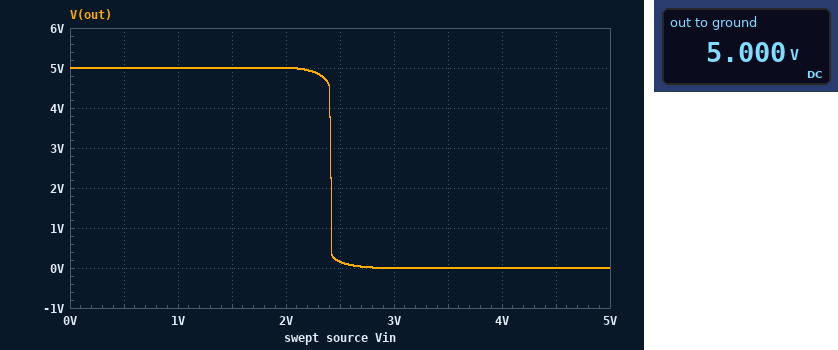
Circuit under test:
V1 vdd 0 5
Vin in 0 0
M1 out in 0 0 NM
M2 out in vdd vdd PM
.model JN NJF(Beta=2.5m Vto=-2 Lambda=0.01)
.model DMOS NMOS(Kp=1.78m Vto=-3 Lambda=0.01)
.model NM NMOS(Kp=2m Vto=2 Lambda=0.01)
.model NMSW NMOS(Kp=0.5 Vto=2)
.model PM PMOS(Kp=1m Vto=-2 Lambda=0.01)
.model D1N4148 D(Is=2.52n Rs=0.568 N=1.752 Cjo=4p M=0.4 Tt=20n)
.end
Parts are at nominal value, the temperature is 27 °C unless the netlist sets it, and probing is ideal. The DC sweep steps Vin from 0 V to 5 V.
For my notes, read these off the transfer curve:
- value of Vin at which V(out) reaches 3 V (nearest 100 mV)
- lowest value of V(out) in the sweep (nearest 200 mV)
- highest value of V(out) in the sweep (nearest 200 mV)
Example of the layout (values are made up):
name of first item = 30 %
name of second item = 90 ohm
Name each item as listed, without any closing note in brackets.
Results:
value of Vin at which V(out) reaches 3 V = 2.4 V
lowest value of V(out) in the sweep = 0 V
highest value of V(out) in the sweep = 5.0 V
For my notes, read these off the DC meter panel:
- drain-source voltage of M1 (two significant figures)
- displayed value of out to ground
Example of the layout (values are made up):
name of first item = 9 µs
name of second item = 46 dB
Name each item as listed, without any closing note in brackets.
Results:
drain-source voltage of M1 = 5.0 V
displayed value of out to ground = 5.000 V
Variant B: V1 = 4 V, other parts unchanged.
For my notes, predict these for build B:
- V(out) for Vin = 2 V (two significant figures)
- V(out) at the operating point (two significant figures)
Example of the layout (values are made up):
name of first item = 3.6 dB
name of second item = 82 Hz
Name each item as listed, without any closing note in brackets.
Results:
V(out) for Vin = 2 V = 2.0 V
V(out) at the operating point = 4.0 V
